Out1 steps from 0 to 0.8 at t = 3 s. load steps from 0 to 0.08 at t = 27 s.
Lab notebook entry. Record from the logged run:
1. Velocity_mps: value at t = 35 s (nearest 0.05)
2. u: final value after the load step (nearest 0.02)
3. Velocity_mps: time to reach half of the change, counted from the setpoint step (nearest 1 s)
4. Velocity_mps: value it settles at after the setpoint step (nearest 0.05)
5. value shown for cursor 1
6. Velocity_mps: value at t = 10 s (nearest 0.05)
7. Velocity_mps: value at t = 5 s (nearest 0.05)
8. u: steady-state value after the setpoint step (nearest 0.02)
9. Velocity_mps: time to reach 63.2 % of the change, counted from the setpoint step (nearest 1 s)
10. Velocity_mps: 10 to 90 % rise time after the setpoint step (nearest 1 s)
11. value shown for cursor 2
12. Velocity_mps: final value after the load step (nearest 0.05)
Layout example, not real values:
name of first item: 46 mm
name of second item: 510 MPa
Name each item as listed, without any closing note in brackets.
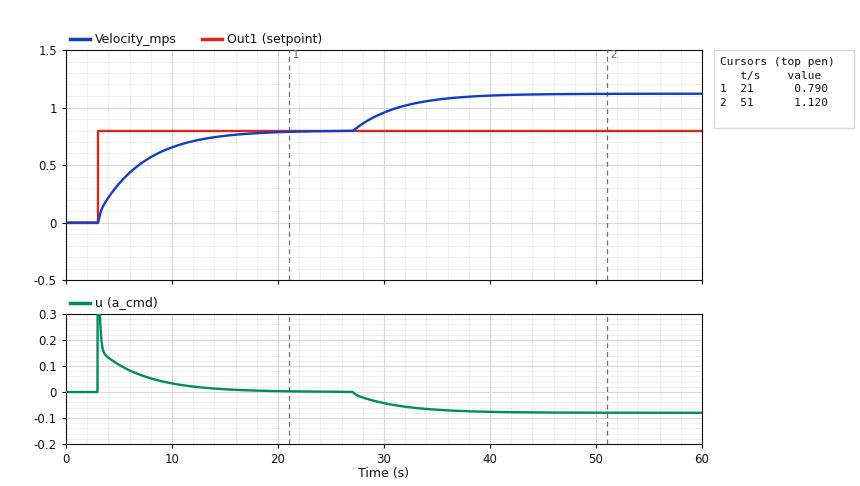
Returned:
Velocity_mps: value at t = 35 s: 1.05
u: final value after the load step: -0.08
Velocity_mps: time to reach half of the change, counted from the setpoint step: 3 s
Velocity_mps: value it settles at after the setpoint step: 0.80
value shown for cursor 1: 0.790
Velocity_mps: value at t = 10 s: 0.65
Velocity_mps: value at t = 5 s: 0.35
u: steady-state value after the setpoint step: 0.00
Velocity_mps: time to reach 63.2 % of the change, counted from the setpoint step: 4 s
Velocity_mps: 10 to 90 % rise time after the setpoint step: 9 s
value shown for cursor 2: 1.120
Velocity_mps: final value after the load step: 1.10
